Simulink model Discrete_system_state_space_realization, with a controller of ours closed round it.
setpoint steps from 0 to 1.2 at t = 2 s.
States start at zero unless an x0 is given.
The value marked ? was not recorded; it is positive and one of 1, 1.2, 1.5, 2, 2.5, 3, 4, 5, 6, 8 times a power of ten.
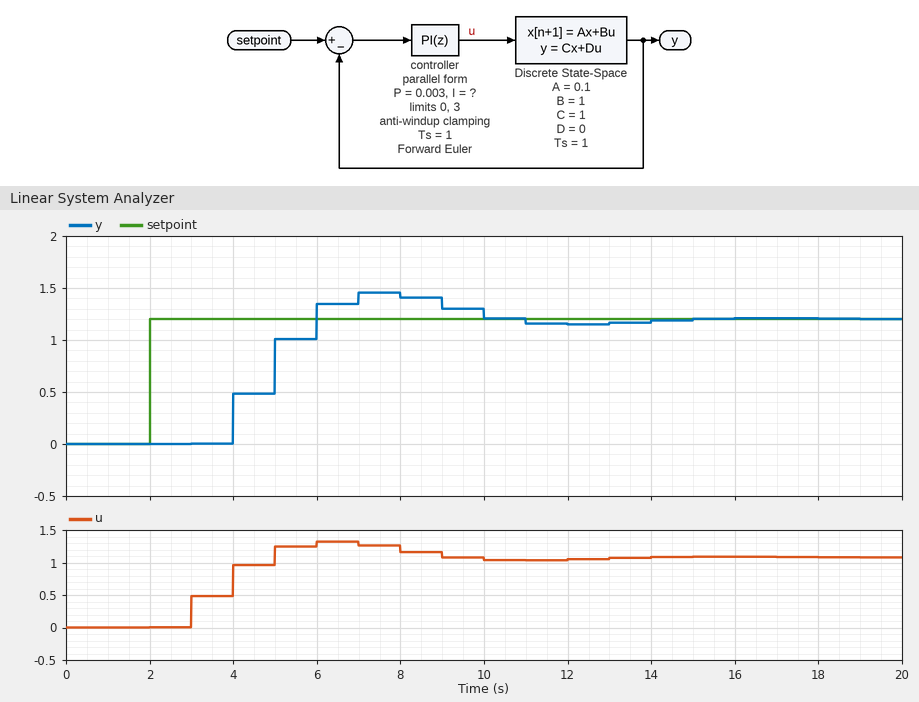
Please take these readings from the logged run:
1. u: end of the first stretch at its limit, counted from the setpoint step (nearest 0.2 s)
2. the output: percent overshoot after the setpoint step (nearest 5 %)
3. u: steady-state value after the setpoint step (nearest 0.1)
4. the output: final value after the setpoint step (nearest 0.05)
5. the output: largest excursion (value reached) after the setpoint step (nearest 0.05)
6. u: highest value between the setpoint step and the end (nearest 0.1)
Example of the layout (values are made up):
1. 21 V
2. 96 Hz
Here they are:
1. 1.0 s
2. 20 %
3. 1.1
4. 1.20
5. 1.45
6. 1.3
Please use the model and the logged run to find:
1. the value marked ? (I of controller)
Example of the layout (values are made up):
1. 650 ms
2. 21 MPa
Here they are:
1. 0.4
